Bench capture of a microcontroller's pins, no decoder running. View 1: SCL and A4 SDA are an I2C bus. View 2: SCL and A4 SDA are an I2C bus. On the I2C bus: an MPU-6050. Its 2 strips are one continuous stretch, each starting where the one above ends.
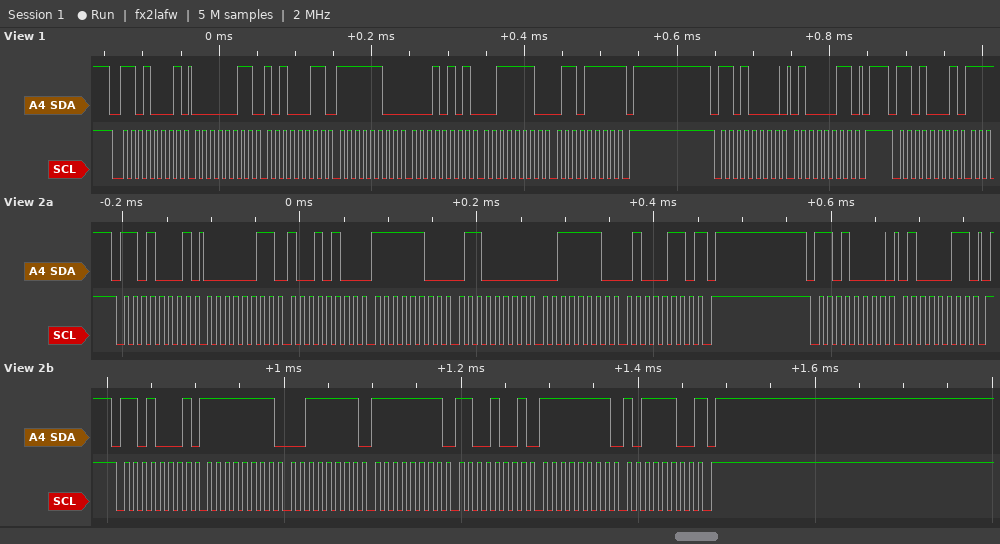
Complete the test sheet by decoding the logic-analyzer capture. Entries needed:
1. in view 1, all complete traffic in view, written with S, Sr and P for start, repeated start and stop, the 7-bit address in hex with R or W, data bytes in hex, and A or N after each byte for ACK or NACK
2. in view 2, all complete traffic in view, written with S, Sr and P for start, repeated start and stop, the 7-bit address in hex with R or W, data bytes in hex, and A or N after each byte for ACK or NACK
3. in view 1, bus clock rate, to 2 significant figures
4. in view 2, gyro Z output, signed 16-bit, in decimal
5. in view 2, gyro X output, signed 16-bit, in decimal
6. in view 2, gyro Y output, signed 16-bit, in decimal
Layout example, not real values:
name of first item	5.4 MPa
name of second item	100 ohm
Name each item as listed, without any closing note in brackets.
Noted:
in view 1, all complete traffic in view, written with S, Sr and P for start, repeated start and stop, the 7-bit address in hex with R or W, data bytes in hex, and A or N after each byte for ACK or NACK	S 68R A 03 A A3 A FC A 15 A 3E A 6F N P S 68W A 43 A P S 68R A
in view 2, all complete traffic in view, written with S, Sr and P for start, repeated start and stop, the 7-bit address in hex with R or W, data bytes in hex, and A or N after each byte for ACK or NACK	S 68R A 03 A 94 A FC A 60 A 3E A 46 N P S 68W A 43 A P S 68R A FF A 3F A FF A C9 A FF A BC N P
in view 1, bus clock rate, to 2 significant figures	100 kHz
in view 2, gyro Z output, signed 16-bit, in decimal	-68
in view 2, gyro X output, signed 16-bit, in decimal	-193
in view 2, gyro Y output, signed 16-bit, in decimal	-55
